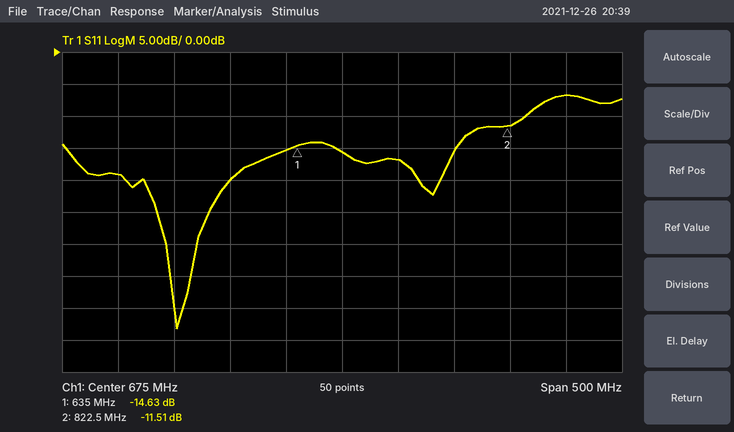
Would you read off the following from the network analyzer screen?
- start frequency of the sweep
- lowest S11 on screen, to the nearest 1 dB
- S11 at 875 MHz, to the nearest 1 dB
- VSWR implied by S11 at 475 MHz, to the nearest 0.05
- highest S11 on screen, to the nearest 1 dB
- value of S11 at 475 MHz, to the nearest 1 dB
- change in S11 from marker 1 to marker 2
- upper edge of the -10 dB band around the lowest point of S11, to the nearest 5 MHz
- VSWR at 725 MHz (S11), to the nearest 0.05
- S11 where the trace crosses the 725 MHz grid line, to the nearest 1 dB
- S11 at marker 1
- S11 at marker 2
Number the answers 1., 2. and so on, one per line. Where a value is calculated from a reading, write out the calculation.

1. 425 MHz
2. -43 dB
3. -7 dB
4. |Γ| = 10^(-19/20) = 0.1122; VSWR = (1 + 0.1122)/(1 − 0.1122) ≈ 1.25
5. -7 dB
6. -19 dB
7. -11.51 − (-14.63) = 3.12 dB
8. 840 MHz
9. |Γ| = 10^(-17/20) = 0.1413; VSWR = (1 + 0.1413)/(1 − 0.1413) ≈ 1.33, so 1.35 to the nearest 0.05
10. -17 dB
11. -14.63 dB
12. -11.51 dB
